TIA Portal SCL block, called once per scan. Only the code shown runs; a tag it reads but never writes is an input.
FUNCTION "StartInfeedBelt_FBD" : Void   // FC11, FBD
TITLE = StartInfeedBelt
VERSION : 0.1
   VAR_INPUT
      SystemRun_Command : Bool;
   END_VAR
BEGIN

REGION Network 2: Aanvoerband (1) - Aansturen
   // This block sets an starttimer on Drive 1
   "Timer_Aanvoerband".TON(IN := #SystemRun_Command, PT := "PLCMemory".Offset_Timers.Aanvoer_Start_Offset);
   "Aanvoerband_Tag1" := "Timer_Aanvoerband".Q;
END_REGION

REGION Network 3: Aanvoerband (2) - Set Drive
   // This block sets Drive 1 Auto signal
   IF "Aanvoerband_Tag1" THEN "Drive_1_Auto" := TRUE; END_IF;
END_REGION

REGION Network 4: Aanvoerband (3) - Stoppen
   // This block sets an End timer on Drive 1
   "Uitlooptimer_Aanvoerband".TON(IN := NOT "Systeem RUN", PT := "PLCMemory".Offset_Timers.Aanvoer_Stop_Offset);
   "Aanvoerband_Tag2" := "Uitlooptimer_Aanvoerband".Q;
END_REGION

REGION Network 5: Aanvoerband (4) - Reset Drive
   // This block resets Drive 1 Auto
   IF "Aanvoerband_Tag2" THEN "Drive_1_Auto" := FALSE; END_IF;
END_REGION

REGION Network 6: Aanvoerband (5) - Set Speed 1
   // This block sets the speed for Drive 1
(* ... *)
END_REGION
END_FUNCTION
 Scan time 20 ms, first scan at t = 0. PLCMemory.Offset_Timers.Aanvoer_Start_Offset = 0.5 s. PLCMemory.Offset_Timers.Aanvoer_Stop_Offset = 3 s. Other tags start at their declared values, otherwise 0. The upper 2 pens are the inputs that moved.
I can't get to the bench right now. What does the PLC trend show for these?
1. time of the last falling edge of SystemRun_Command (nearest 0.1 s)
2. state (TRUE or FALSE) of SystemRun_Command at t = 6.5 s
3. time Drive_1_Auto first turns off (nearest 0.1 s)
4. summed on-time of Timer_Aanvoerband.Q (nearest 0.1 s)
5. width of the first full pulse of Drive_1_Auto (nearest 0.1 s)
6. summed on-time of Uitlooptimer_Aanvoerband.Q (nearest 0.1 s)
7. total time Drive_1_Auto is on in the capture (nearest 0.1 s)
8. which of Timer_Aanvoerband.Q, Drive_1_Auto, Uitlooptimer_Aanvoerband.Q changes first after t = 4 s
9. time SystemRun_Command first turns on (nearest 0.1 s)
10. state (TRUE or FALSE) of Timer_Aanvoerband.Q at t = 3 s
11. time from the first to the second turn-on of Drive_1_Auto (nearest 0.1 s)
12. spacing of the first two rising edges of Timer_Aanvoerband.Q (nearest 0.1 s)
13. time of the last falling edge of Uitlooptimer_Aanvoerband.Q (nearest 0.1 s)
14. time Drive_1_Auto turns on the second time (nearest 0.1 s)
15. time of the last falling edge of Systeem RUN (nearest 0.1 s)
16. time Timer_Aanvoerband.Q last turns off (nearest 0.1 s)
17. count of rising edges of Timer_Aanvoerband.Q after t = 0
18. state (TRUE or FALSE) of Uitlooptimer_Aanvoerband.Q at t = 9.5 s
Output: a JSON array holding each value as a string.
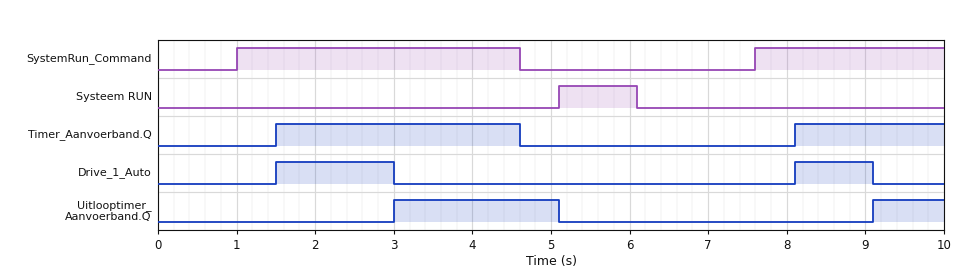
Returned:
["4.6 s", "FALSE", "3.0 s", "5.0 s", "1.5 s", "3.0 s", "2.5 s", "Timer_Aanvoerband.Q", "1.0 s", "TRUE", "6.6 s", "6.6 s", "5.1 s", "8.1 s", "6.1 s", "4.6 s", "2", "TRUE"]
